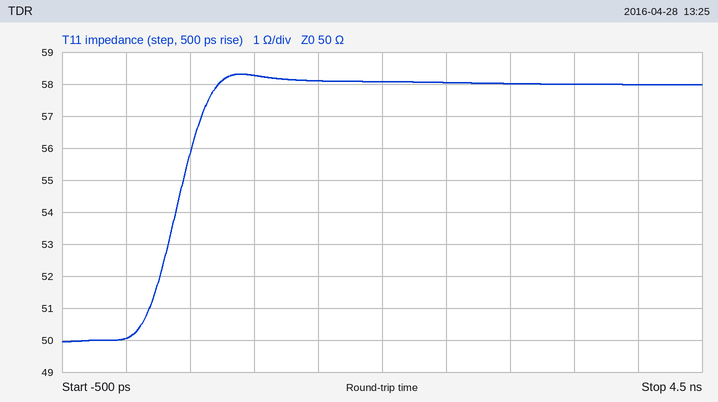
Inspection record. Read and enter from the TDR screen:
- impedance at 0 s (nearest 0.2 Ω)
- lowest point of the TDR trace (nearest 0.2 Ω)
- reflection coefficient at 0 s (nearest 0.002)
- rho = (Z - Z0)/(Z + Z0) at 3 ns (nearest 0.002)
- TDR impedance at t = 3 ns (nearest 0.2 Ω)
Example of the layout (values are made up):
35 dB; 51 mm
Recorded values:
50.0 Ω; 50.0 Ω; 0.000; +0.074; 58.0 Ω
